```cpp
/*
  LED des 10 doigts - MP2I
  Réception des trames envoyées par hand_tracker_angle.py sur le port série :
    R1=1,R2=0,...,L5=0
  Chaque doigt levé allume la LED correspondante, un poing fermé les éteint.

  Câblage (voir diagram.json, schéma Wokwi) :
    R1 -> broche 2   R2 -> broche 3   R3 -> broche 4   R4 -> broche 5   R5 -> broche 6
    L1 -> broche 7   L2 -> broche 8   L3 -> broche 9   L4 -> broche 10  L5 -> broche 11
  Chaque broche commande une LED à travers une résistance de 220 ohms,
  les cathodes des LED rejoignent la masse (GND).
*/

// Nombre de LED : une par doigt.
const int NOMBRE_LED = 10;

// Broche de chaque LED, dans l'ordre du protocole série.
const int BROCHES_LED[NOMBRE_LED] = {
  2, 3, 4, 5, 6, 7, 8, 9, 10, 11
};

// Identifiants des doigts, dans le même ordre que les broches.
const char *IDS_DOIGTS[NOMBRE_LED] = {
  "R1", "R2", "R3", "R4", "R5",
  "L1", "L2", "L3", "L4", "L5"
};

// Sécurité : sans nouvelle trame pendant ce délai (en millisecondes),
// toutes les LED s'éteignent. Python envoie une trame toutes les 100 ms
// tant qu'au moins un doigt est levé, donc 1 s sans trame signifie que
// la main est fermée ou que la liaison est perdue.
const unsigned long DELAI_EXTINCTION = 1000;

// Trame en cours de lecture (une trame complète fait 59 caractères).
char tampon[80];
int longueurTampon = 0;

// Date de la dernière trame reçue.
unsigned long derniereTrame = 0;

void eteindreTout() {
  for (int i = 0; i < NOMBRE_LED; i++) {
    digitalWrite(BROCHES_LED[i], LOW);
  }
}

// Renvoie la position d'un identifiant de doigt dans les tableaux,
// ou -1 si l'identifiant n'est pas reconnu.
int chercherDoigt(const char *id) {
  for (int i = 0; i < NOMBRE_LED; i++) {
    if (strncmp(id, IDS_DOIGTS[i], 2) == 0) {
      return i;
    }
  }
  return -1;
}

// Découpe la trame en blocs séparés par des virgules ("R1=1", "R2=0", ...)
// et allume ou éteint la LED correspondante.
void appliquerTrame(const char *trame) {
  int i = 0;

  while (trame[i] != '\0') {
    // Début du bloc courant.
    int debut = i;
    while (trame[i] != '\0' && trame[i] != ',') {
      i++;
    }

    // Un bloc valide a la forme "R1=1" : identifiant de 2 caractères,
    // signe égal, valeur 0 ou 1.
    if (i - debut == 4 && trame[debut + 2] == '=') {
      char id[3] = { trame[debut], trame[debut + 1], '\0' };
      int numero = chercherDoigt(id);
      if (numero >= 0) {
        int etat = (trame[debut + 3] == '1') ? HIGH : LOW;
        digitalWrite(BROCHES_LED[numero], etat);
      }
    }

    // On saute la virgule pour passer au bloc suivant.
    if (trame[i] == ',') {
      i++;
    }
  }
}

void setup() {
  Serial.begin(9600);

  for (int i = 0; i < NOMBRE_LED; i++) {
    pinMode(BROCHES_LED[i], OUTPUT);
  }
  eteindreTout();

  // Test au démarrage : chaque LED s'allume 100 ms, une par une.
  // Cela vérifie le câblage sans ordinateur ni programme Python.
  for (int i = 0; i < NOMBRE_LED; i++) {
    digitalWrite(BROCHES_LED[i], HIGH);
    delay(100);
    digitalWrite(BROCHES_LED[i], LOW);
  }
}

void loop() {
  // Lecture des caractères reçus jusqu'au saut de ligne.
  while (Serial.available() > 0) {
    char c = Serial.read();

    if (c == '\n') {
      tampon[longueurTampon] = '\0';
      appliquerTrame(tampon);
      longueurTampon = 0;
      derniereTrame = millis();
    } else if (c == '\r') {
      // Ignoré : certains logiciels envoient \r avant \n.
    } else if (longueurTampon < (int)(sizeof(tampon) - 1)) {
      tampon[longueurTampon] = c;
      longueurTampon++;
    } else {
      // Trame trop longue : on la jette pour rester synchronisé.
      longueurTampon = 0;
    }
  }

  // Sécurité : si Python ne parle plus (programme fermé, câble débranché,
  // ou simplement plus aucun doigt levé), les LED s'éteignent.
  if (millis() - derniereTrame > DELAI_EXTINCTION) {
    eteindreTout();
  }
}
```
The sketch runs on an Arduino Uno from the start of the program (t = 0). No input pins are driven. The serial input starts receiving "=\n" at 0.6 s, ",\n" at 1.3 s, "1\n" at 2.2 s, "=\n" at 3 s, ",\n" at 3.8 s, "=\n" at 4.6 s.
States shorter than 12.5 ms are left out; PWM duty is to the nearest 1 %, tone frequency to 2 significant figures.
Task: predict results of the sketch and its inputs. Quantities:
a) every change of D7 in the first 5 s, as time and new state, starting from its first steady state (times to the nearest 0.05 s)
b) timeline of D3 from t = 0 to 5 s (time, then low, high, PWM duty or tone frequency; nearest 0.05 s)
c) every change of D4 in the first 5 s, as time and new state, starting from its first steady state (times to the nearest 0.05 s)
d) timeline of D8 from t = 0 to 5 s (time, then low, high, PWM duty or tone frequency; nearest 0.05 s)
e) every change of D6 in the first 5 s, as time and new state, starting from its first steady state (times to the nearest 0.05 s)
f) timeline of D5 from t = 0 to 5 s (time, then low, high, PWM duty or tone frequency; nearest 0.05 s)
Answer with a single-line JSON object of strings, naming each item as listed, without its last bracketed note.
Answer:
{"every change of D7 in the first 5 s, as time and new state, starting from its first steady state": "0 s low; 0.5 s high; 0.6 s low", "timeline of D3 from t = 0 to 5 s": "0 s low; 0.1 s high; 0.2 s low", "every change of D4 in the first 5 s, as time and new state, starting from its first steady state": "0 s low; 0.2 s high; 0.3 s low", "timeline of D8 from t = 0 to 5 s": "0 s low; 0.6 s high; 0.7 s low", "every change of D6 in the first 5 s, as time and new state, starting from its first steady state": "0 s low; 0.4 s high; 0.5 s low", "timeline of D5 from t = 0 to 5 s": "0 s low; 0.3 s high; 0.4 s low"}
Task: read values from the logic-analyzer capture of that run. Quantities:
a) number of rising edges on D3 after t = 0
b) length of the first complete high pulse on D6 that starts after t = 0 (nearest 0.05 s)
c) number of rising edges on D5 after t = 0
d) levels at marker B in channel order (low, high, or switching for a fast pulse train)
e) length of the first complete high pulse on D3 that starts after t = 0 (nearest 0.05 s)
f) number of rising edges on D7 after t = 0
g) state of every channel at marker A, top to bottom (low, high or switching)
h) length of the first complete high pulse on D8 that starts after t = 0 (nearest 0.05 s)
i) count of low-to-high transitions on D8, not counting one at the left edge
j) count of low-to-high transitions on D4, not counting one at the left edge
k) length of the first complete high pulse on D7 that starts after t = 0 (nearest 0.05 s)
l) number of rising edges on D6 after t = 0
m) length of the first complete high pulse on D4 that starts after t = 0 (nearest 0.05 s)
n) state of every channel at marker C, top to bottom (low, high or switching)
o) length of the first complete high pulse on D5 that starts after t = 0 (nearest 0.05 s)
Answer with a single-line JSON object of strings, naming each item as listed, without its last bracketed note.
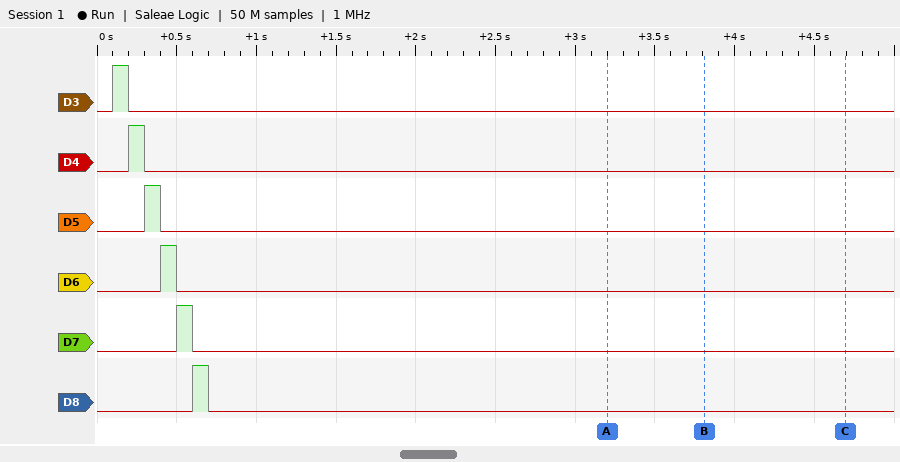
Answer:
{"number of rising edges on D3 after t = 0": "1", "length of the first complete high pulse on D6 that starts after t = 0": "0.10 s", "number of rising edges on D5 after t = 0": "1", "levels at marker B in channel order": "D3 low, D4 low, D5 low, D6 low, D7 low, D8 low", "length of the first complete high pulse on D3 that starts after t = 0": "0.10 s", "number of rising edges on D7 after t = 0": "1", "state of every channel at marker A, top to bottom": "D3 low, D4 low, D5 low, D6 low, D7 low, D8 low", "length of the first complete high pulse on D8 that starts after t = 0": "0.10 s", "count of low-to-high transitions on D8, not counting one at the left edge": "1", "count of low-to-high transitions on D4, not counting one at the left edge": "1", "length of the first complete high pulse on D7 that starts after t = 0": "0.10 s", "number of rising edges on D6 after t = 0": "1", "length of the first complete high pulse on D4 that starts after t = 0": "0.10 s", "state of every channel at marker C, top to bottom": "D3 low, D4 low, D5 low, D6 low, D7 low, D8 low", "length of the first complete high pulse on D5 that starts after t = 0": "0.10 s"}
